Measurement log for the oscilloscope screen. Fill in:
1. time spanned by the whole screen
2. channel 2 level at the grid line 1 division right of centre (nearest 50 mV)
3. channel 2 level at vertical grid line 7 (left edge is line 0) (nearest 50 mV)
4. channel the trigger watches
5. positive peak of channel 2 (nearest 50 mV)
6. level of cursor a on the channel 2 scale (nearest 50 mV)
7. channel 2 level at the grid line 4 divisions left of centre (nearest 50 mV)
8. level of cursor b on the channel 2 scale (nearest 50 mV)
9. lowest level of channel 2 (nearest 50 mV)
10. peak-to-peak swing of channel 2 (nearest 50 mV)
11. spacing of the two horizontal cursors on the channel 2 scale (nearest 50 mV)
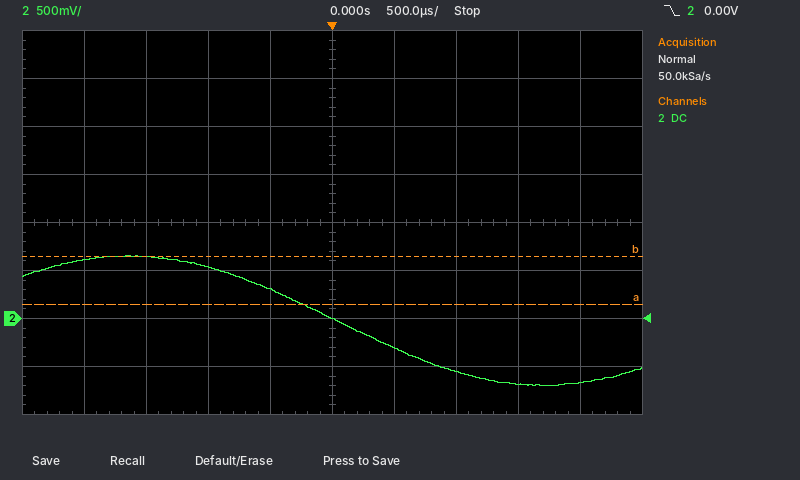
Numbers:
5 ms
-300 mV
-550 mV
channel 2
650 mV
150 mV
600 mV
650 mV
-700 mV
1.35 V
500 mV
